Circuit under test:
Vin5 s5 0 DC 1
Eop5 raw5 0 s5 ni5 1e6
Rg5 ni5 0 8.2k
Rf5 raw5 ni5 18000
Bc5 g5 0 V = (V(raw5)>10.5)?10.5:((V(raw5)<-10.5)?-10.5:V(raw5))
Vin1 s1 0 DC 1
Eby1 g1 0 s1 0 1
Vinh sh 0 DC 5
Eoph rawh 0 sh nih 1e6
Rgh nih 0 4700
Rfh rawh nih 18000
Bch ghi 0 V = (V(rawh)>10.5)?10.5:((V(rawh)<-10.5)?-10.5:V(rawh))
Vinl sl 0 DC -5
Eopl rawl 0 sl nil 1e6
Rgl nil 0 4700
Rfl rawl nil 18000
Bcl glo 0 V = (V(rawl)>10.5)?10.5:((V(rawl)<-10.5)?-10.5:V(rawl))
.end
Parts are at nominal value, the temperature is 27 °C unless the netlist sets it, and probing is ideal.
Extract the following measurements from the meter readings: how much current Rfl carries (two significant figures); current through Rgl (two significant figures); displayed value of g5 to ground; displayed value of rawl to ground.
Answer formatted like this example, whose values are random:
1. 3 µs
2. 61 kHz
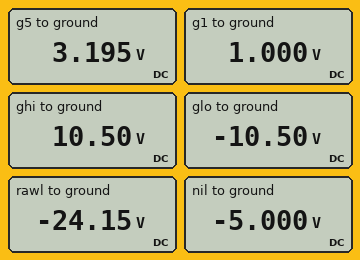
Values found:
1. 1.1 mA
2. 1.1 mA
3. 3.195 V
4. -24.15 V
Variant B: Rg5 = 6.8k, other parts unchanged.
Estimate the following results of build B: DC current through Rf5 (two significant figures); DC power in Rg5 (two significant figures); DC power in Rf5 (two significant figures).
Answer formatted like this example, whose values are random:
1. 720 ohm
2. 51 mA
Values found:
1. 150 µA
2. 150 µW
3. 390 µW
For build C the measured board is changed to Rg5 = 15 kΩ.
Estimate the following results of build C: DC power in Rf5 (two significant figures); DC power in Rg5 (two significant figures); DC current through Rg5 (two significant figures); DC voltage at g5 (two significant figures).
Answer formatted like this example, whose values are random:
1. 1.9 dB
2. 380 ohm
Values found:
1. 80 µW
2. 67 µW
3. 67 µA
4. 2.2 V
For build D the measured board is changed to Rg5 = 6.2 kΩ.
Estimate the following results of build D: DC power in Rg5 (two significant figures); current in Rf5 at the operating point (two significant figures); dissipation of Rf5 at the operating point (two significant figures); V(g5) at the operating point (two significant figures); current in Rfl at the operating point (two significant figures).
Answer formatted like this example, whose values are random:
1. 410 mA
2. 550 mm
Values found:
1. 160 µW
2. 160 µA
3. 470 µW
4. 3.9 V
5. 1.1 mA
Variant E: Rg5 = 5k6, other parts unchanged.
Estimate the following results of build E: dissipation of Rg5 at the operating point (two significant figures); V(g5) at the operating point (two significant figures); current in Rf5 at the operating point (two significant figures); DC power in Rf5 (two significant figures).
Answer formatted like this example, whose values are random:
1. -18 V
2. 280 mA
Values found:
1. 180 µW
2. 4.2 V
3. 180 µA
4. 570 µW
